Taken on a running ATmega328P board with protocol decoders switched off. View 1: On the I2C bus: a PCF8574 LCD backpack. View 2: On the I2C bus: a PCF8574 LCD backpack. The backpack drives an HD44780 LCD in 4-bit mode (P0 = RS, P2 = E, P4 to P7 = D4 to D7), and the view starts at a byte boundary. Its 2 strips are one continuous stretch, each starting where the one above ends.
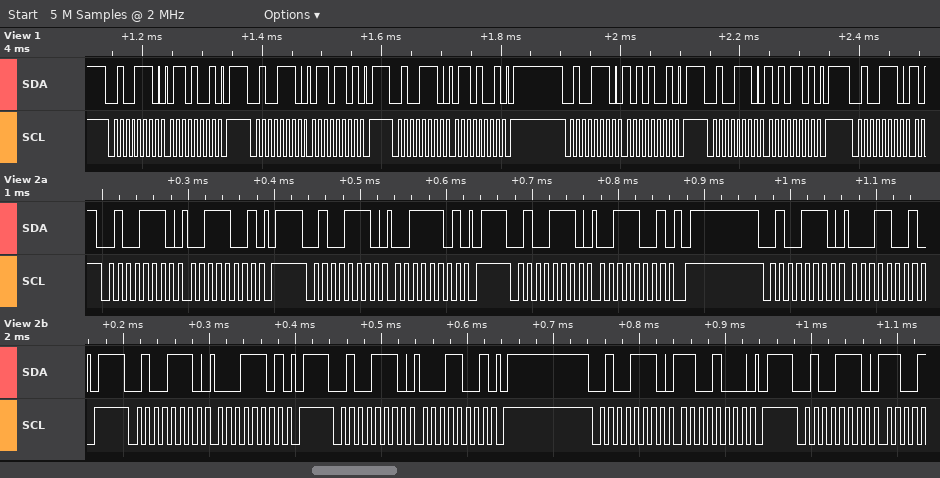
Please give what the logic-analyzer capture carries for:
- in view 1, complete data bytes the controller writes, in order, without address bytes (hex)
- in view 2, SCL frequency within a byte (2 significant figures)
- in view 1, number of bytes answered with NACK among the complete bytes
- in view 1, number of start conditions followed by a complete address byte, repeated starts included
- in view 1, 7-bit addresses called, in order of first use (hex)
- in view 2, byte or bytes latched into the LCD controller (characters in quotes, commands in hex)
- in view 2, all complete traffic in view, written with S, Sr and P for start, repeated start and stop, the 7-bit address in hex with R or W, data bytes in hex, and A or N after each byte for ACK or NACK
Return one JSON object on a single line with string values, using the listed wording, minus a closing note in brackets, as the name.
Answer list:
{"in view 1, complete data bytes the controller writes, in order, without address bytes": "69 6D 69 A9 AD", "in view 2, SCL frequency within a byte": "100 kHz", "in view 1, number of bytes answered with NACK among the complete bytes": "0", "in view 1, number of start conditions followed by a complete address byte, repeated starts included": "6", "in view 1, 7-bit addresses called, in order of first use": "0x27", "in view 2, byte or bytes latched into the LCD controller": "'1'", "in view 2, all complete traffic in view, written with S, Sr and P for start, repeated start and stop, the 7-bit address in hex with R or W, data bytes in hex, and A or N after each byte for ACK or NACK": "S 27W A 39 A P S 27W A 3D A P S 27W A 39 A P S 27W A 19 A P S 27W A 1D A P S 27W A 19 A P S 27W A C8 A P S 27W A"}
